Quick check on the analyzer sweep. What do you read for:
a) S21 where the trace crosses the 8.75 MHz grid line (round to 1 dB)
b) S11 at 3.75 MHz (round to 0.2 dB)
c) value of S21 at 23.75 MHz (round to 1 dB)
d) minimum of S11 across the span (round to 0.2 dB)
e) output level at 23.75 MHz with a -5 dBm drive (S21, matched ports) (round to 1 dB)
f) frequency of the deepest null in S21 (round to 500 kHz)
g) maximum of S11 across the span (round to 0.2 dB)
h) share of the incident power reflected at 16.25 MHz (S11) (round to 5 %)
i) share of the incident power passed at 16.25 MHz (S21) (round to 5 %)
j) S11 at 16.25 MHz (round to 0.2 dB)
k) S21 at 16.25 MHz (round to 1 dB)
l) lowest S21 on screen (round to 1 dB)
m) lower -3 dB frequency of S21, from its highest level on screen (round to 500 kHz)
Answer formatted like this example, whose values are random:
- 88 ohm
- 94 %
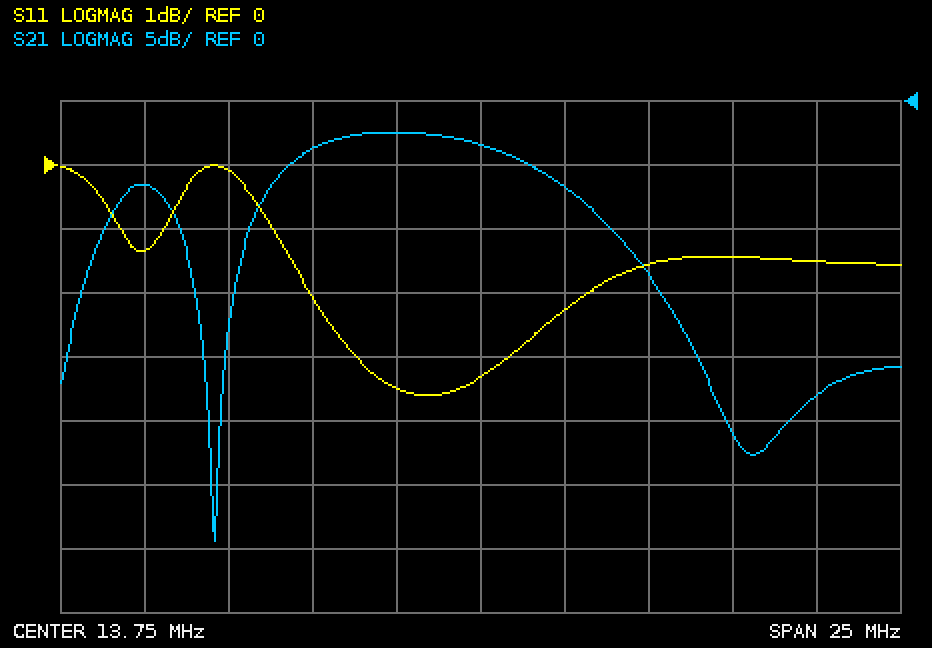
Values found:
- -4 dB
- -1.4 dB
- -23 dB
- -3.6 dB
- -28 dBm
- 6.0 MHz
- 0.0 dB
- 60 %
- 20 %
- -2.2 dB
- -7 dB
- -34 dB
- 8.0 MHz
